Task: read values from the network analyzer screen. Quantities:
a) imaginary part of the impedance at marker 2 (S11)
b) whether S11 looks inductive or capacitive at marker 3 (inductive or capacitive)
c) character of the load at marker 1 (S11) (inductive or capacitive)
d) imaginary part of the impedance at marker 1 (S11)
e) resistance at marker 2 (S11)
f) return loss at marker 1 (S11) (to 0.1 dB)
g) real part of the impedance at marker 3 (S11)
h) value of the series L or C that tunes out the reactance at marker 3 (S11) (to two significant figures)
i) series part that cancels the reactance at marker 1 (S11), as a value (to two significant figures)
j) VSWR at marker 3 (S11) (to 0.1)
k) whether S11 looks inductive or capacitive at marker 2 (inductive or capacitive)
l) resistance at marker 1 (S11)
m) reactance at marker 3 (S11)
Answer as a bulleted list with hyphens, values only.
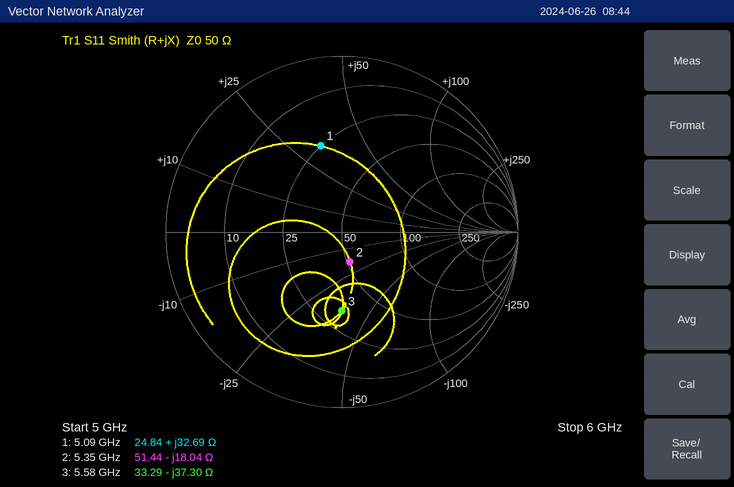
- -18.04 Ω
- capacitive
- inductive
- +32.69 Ω
- 51.44 Ω
- 5.9 dB
- 33.29 Ω
- 1.1 nH
- 960 fF
- 2.6
- capacitive
- 24.84 Ω
- -37.30 Ω
